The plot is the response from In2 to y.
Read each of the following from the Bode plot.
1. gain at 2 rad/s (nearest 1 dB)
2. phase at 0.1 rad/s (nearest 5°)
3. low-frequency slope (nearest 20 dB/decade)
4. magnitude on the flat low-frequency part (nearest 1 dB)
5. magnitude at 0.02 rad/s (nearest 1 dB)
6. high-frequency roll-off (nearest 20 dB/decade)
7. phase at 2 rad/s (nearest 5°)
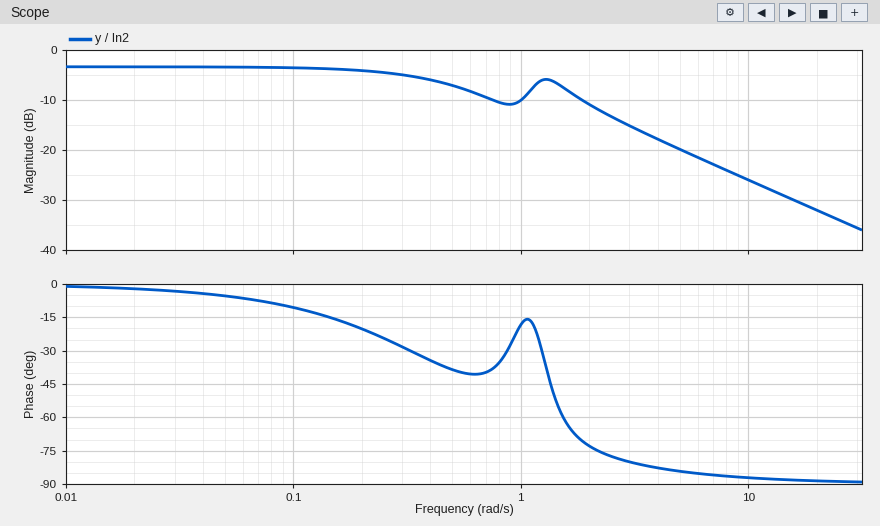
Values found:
-11 dB
-10°
0 dB/decade
-3 dB
-3 dB
-20 dB/decade
-75°
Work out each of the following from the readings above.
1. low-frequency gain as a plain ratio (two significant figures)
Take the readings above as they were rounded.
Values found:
0.71
